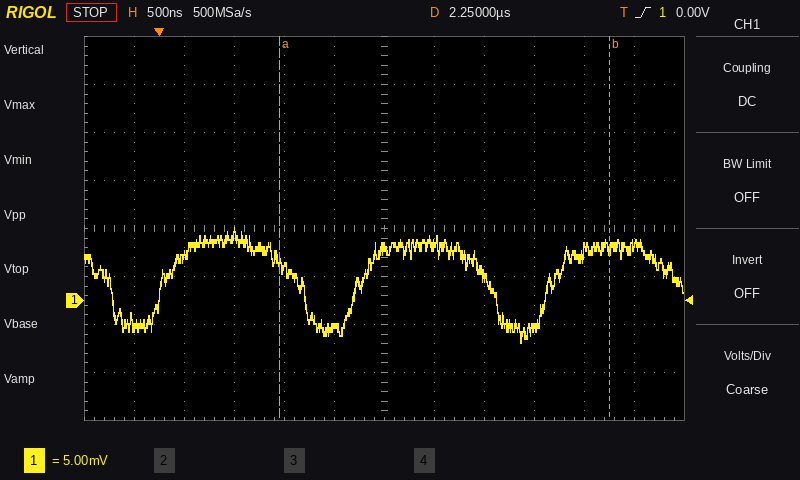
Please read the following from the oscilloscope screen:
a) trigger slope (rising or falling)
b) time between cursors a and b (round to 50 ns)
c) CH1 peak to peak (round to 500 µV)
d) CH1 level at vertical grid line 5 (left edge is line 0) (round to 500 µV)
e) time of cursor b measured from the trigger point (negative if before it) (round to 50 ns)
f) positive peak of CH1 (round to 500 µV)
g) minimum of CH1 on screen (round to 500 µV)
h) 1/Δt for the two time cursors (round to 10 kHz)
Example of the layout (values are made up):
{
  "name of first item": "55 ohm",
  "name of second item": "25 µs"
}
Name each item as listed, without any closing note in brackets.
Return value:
{
  "trigger slope": "rising",
  "time between cursors a and b": "3.30 µs",
  "CH1 peak to peak": "12.0 mV",
  "CH1 level at vertical grid line 5 (left edge is line 0)": "-3.0 mV",
  "time of cursor b measured from the trigger point (negative if before it)": "+4.50 µs",
  "positive peak of CH1": "7.5 mV",
  "minimum of CH1 on screen": "-4.5 mV",
  "1/Δt for the two time cursors": "300 kHz"
}
